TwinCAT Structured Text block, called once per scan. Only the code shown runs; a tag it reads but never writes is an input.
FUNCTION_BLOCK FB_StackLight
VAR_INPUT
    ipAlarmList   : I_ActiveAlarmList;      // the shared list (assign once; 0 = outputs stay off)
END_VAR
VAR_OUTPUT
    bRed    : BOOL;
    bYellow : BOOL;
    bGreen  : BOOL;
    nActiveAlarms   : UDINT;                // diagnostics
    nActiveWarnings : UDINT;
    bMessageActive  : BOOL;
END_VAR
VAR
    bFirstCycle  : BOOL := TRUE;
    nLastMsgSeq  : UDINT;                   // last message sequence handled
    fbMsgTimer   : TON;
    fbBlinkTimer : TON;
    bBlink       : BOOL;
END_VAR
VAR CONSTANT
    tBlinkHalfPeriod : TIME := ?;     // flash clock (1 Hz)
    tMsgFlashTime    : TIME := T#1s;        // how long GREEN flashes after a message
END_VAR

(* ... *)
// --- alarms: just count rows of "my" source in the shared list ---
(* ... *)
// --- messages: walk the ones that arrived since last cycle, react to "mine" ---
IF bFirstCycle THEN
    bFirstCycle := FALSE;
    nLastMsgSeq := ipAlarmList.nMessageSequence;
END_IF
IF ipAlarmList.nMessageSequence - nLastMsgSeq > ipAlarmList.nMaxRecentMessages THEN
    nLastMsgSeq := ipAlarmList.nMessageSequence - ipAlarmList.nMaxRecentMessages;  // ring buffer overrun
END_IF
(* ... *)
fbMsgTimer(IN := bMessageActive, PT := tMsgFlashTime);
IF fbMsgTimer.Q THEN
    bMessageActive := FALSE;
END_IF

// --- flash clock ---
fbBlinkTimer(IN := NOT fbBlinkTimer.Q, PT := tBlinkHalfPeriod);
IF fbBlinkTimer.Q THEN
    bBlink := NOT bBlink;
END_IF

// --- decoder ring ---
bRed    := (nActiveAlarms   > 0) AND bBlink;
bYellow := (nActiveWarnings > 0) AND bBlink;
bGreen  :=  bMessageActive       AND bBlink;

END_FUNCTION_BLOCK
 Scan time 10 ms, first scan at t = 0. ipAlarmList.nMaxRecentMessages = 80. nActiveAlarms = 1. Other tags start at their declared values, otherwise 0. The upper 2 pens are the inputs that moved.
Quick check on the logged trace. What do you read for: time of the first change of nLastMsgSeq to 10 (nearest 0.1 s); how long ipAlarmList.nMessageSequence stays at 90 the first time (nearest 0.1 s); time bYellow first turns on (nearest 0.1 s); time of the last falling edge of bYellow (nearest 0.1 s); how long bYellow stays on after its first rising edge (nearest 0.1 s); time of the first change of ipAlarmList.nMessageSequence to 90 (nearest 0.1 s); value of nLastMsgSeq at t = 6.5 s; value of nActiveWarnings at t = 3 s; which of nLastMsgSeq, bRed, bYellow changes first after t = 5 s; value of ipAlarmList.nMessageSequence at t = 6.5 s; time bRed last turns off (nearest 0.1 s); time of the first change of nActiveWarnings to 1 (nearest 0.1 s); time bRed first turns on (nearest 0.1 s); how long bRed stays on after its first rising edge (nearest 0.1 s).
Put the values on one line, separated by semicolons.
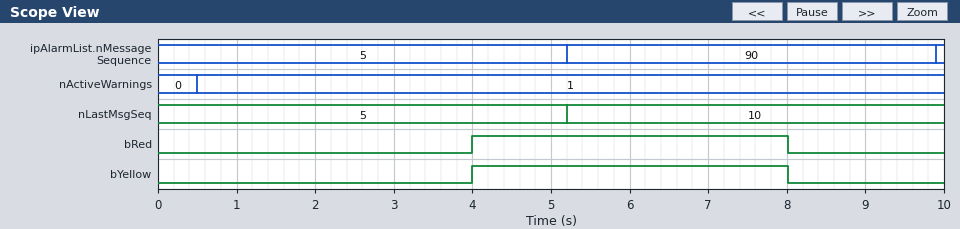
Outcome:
5.2 s; 4.7 s; 4.0 s; 8.0 s; 4.0 s; 5.2 s; 10; 1; nLastMsgSeq; 90; 8.0 s; 0.5 s; 4.0 s; 4.0 s
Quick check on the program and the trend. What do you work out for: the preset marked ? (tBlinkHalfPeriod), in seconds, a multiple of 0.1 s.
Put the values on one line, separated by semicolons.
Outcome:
4.0 s
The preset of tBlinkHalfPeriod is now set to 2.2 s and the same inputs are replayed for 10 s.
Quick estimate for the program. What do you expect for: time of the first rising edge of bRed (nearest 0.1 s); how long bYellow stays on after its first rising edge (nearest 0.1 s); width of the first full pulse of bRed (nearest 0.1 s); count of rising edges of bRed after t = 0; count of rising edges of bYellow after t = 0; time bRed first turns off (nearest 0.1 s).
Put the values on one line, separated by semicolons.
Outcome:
2.2 s; 2.2 s; 2.2 s; 2; 2; 4.4 s
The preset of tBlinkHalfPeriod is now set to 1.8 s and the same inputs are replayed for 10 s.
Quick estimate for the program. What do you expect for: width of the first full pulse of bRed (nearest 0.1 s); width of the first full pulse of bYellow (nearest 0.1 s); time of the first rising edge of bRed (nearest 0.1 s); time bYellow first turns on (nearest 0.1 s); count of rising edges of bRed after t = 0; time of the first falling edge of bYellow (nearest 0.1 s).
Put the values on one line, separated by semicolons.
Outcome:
1.8 s; 1.8 s; 1.8 s; 1.8 s; 3; 3.6 s
